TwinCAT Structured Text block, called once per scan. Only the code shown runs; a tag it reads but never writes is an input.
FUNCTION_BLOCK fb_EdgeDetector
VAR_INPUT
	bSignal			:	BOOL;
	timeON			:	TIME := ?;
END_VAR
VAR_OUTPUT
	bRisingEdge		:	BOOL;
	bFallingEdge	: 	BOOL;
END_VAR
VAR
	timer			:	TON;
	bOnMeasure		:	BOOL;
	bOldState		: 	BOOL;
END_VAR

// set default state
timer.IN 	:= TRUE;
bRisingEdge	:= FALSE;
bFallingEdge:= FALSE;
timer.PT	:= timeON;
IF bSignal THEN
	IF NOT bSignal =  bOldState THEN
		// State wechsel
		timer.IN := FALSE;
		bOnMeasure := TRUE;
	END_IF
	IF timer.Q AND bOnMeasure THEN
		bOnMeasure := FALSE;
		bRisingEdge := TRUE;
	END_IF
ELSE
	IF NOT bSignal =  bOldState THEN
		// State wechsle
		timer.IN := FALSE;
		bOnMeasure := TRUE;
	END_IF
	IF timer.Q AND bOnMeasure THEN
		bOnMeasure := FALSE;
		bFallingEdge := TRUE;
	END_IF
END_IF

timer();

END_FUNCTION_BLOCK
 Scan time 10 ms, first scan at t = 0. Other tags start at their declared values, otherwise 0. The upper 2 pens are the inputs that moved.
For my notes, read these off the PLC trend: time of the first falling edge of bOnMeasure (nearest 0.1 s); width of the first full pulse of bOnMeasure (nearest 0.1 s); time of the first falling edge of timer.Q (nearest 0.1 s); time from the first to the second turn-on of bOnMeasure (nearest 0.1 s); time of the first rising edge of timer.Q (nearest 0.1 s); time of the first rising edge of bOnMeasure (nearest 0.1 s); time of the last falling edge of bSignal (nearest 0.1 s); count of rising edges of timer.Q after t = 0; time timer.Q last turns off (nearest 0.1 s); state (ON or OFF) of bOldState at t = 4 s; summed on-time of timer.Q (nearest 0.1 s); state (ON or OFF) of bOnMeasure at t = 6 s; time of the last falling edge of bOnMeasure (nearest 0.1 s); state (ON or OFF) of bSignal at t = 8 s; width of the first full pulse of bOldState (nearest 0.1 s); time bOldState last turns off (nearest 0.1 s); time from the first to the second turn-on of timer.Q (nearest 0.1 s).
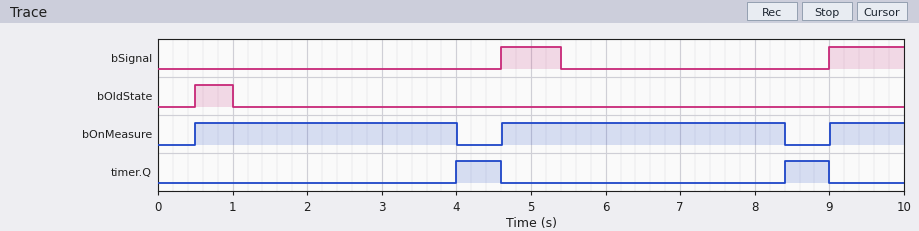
4.0 s
3.5 s
4.6 s
4.1 s
4.0 s
0.5 s
5.4 s
2
9.0 s
OFF
1.2 s
ON
8.4 s
OFF
0.5 s
1.0 s
4.4 s
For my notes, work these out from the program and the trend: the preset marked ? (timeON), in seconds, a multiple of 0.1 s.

3.0 s
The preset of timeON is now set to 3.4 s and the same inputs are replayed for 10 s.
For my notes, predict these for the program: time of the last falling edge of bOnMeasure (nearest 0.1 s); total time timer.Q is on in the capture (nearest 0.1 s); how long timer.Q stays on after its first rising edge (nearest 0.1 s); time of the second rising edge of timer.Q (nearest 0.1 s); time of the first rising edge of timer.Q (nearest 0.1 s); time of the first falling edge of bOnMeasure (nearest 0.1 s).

8.8 s
0.4 s
0.2 s
8.8 s
4.4 s
4.4 s
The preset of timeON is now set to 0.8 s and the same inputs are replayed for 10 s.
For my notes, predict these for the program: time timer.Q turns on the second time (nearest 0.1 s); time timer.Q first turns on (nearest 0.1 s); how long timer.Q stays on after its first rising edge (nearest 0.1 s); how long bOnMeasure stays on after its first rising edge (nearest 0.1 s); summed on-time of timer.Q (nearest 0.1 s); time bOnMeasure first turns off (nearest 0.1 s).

6.2 s
1.8 s
2.8 s
1.3 s
5.6 s
1.8 s
